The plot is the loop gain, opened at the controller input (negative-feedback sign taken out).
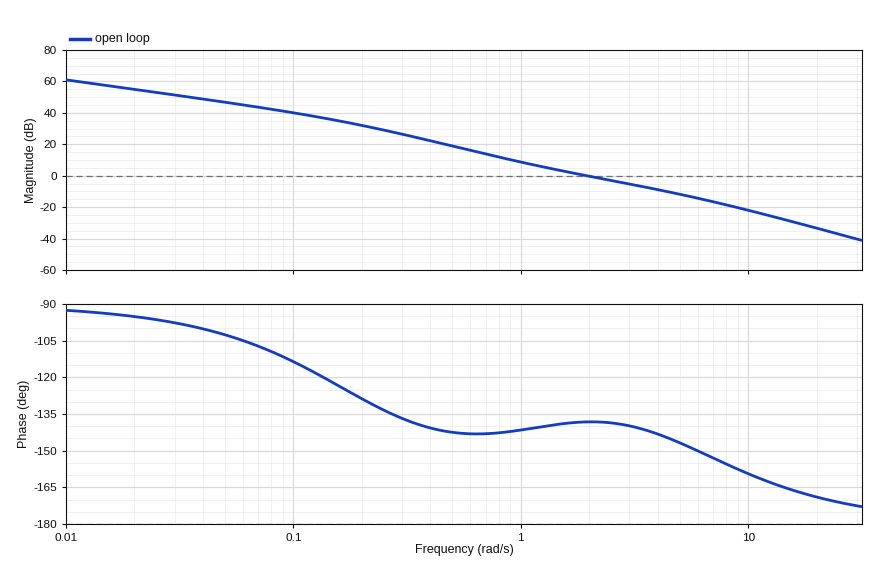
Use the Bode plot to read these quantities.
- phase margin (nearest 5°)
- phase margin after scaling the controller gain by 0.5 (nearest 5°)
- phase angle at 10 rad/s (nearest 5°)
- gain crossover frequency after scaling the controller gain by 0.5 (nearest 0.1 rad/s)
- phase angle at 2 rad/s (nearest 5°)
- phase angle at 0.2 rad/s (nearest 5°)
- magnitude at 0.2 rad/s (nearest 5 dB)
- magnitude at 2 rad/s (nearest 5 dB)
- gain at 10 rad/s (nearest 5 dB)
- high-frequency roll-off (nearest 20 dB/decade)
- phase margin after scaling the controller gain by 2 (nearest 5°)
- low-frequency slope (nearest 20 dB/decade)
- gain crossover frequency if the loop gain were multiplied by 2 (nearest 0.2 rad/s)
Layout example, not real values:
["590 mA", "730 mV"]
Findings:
["40°", "40°", "-160°", "1.2 rad/s", "-140°", "-130°", "30 dB", "0 dB", "-20 dB", "-40 dB/decade", "40°", "-20 dB/decade", "3.2 rad/s"]
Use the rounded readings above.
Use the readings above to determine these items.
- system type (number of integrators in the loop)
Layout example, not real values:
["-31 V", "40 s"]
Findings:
["1"]
